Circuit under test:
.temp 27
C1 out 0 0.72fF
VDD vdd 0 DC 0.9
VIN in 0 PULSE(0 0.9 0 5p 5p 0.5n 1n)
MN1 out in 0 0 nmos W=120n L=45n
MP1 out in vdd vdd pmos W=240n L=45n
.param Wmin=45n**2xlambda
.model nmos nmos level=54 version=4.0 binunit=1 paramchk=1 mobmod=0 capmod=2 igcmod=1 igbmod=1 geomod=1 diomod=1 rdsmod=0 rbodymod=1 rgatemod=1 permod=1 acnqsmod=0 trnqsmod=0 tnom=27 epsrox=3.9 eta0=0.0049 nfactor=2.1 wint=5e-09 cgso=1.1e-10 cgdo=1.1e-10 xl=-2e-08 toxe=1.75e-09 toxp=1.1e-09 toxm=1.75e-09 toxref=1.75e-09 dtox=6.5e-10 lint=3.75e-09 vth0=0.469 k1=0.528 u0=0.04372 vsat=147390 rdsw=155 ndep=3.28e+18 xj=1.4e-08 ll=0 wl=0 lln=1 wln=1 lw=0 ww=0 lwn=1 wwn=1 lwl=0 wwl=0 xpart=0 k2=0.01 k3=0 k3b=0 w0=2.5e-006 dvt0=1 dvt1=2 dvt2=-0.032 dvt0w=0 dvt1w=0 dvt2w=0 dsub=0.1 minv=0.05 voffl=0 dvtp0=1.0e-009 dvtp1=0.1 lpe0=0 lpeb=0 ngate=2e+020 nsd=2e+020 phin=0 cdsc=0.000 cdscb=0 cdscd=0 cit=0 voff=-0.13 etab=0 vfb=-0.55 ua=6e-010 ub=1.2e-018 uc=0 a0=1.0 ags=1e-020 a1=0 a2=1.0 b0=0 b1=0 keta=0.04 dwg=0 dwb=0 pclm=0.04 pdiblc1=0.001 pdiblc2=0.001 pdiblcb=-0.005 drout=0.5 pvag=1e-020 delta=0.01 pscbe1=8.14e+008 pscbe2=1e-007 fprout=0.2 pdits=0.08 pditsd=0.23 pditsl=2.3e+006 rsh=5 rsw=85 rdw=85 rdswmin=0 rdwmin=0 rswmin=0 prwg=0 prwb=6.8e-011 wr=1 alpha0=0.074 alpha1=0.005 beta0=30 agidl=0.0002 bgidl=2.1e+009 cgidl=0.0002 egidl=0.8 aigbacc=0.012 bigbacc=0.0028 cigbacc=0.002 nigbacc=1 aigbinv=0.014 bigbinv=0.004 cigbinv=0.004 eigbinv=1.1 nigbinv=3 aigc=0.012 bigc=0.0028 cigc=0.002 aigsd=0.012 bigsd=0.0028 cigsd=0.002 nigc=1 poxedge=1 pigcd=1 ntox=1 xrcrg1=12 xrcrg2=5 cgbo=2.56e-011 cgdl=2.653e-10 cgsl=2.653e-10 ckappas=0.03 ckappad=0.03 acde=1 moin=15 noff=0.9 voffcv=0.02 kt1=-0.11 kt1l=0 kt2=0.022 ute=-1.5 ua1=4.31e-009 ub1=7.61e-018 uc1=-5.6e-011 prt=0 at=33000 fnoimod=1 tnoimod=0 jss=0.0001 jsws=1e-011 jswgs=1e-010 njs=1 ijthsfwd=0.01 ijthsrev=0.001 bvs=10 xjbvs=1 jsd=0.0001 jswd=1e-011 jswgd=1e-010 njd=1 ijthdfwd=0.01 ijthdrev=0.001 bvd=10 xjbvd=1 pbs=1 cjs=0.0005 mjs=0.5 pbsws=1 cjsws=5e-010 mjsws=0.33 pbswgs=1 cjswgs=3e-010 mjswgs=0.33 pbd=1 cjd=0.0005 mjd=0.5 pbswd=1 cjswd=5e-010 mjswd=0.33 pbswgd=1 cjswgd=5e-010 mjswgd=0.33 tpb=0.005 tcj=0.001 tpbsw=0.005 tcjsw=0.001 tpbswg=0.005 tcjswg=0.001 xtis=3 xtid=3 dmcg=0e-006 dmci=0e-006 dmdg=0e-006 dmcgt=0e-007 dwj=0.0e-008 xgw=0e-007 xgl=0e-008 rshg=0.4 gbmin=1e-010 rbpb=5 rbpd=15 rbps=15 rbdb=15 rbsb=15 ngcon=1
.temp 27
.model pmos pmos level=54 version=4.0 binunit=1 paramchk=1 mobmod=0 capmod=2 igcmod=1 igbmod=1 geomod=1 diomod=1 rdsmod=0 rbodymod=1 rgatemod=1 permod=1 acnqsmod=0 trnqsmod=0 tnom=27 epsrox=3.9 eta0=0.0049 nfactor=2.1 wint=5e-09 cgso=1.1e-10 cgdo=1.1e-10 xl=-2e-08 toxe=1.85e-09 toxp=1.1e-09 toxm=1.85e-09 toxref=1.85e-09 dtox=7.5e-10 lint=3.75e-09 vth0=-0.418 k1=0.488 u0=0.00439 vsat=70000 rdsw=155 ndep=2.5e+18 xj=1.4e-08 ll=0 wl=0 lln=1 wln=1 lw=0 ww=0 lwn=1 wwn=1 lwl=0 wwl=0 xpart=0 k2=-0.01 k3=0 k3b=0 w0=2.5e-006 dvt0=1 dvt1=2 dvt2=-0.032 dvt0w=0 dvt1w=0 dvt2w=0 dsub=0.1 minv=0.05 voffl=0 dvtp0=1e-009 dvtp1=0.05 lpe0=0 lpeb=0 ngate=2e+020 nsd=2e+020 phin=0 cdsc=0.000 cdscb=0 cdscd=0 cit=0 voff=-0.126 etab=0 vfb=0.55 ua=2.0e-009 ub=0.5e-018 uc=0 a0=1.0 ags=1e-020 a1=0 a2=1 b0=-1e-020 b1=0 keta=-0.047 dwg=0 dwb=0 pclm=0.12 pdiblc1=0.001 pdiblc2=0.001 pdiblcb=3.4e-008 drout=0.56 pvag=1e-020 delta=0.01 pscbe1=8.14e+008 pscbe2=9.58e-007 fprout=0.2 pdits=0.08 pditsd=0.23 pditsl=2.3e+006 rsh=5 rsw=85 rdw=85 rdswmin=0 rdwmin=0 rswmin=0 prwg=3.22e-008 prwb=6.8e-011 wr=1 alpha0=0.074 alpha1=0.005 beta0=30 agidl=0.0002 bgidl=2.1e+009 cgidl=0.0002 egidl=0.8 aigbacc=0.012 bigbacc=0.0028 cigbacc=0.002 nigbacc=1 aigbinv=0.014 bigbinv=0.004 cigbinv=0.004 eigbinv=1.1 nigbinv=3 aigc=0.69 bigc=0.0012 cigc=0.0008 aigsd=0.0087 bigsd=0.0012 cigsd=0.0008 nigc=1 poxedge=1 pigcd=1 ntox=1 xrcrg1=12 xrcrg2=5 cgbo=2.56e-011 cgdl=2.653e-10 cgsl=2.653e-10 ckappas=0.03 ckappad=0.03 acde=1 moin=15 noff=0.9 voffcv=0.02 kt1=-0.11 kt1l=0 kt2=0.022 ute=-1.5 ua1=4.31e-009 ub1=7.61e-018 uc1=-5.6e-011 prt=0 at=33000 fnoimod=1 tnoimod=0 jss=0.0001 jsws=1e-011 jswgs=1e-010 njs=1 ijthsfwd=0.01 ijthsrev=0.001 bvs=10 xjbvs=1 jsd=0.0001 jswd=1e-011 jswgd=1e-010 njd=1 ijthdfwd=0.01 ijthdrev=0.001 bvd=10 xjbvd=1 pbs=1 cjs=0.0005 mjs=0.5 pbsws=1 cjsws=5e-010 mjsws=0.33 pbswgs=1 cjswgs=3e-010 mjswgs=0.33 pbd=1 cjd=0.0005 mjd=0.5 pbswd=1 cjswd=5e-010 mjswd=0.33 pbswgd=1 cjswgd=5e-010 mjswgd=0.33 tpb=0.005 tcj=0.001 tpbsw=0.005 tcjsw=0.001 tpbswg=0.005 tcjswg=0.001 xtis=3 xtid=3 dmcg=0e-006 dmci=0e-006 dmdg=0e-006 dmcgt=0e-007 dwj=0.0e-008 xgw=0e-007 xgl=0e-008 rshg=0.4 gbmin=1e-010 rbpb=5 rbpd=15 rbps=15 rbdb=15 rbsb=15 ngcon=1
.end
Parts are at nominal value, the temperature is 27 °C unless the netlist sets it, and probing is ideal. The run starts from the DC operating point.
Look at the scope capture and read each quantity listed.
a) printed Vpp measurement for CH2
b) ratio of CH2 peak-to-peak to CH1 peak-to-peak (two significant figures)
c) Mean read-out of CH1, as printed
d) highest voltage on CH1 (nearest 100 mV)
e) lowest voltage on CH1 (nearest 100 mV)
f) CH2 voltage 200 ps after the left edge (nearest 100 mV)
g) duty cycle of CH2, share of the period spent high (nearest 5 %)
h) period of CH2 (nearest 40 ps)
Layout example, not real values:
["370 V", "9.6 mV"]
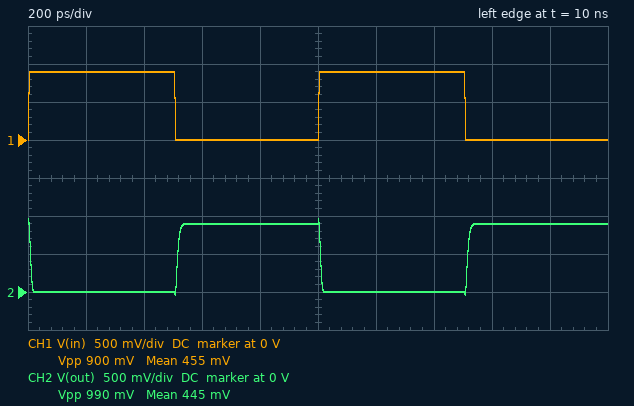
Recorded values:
["990 mV", "1.1", "455 mV", "900 mV", "0 V", "0 V", "50 %", "1.00 ns"]
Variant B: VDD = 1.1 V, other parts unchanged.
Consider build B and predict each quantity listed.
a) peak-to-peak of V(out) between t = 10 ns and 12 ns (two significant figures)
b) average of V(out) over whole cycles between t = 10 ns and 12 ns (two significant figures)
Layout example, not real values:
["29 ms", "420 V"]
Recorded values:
["1.2 V", "550 mV"]
